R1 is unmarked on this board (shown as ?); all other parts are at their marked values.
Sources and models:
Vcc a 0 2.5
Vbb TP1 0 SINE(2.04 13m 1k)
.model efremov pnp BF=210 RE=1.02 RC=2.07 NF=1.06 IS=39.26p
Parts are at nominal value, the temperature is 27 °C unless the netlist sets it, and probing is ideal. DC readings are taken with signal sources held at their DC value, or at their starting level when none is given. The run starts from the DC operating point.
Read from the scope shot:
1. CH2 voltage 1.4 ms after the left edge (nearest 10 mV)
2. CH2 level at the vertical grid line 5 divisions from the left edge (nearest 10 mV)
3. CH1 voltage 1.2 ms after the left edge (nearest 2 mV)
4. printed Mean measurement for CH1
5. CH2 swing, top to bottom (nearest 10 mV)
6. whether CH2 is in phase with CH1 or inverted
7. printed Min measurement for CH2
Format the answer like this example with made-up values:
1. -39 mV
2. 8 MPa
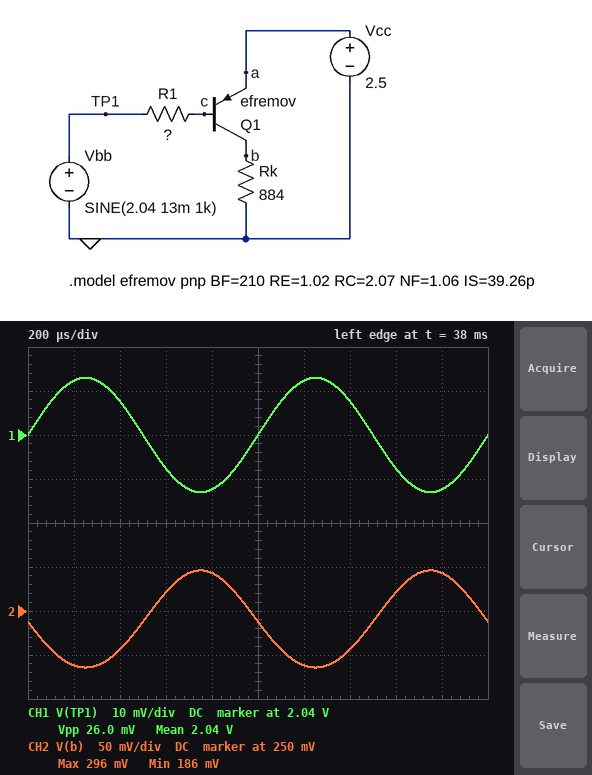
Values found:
1. 210 mV
2. 240 mV
3. 2.052 V
4. 2.04 V
5. 110 mV
6. inverted
7. 186 mV
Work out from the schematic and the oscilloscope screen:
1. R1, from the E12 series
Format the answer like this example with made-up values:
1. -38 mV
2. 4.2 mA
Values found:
1. 22 kΩ
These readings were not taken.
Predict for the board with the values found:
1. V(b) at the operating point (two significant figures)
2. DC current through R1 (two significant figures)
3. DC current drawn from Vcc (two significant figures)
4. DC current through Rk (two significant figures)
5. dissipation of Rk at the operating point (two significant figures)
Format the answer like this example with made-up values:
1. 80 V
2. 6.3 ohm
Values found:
1. 240 mV
2. 1.3 µA
3. 270 µA
4. 270 µA
5. 64 µW
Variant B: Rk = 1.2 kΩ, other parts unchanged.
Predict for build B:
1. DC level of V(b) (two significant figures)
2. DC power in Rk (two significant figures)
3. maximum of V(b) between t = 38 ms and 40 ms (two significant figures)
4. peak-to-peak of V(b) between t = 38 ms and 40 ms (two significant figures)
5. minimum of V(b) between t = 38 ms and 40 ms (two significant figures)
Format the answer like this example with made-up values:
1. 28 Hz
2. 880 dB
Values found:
1. 320 mV
2. 87 µW
3. 400 mV
4. 150 mV
5. 250 mV
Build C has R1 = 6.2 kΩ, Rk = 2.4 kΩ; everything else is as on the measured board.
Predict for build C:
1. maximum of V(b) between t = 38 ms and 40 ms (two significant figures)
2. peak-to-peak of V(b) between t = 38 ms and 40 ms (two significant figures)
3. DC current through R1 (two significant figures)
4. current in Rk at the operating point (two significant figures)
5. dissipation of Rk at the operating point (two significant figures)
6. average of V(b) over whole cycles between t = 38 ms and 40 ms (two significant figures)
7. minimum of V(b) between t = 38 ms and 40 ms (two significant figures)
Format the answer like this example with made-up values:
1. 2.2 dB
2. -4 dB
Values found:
1. 1.5 V
2. 690 mV
3. 2.2 µA
4. 460 µA
5. 500 µW
6. 1.1 V
7. 790 mV
